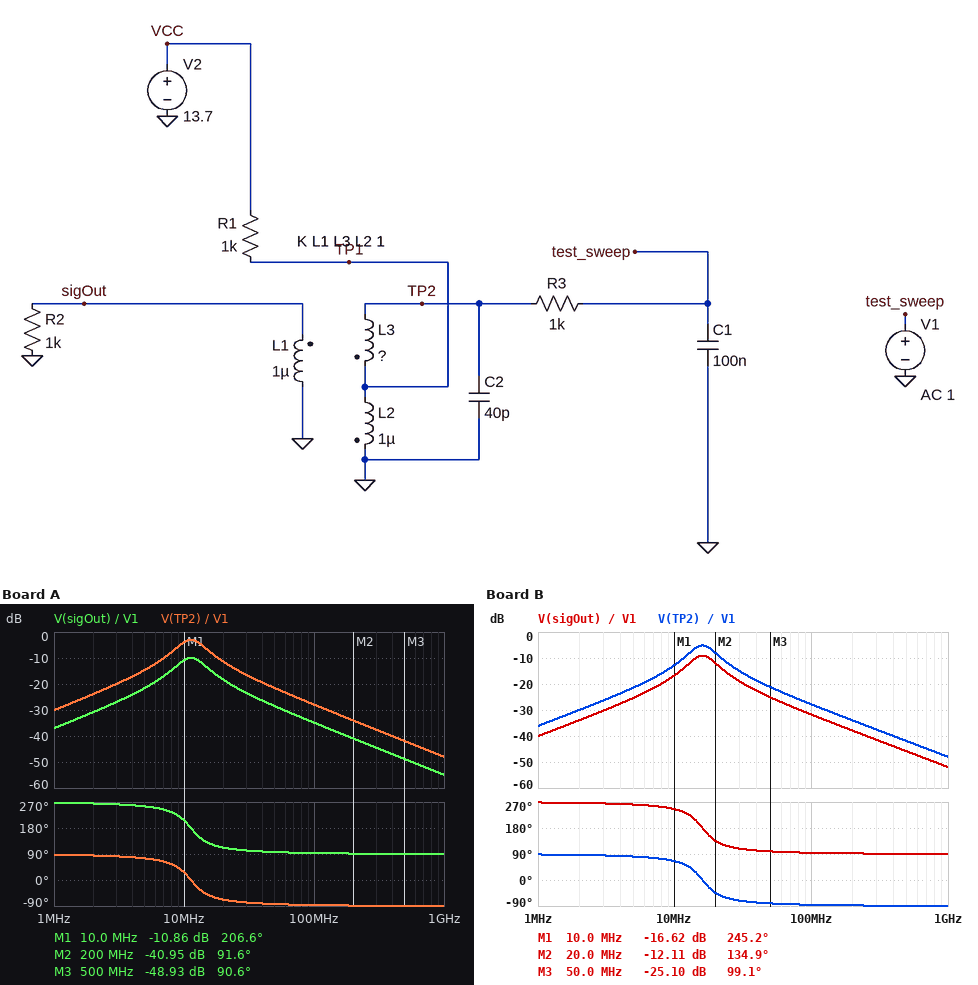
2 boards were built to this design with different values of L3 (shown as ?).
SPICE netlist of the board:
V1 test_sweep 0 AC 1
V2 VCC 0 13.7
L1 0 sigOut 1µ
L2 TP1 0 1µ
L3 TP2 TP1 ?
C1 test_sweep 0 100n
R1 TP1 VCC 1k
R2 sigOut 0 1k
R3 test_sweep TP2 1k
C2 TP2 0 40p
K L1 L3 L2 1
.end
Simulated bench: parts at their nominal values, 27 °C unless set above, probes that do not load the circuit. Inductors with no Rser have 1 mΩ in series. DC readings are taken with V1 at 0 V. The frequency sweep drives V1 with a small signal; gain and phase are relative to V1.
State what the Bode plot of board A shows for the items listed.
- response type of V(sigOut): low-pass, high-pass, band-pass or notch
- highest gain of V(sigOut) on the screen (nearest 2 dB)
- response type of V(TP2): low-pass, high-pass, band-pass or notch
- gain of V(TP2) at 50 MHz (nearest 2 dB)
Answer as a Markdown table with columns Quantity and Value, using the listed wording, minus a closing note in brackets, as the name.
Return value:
| Quantity | Value |
|---|---|
| response type of V(sigOut): low-pass, high-pass, band-pass or notch | band-pass |
| highest gain of V(sigOut) on the screen | -10 dB |
| response type of V(TP2): low-pass, high-pass, band-pass or notch | band-pass |
| gain of V(TP2) at 50 MHz | -22 dB |
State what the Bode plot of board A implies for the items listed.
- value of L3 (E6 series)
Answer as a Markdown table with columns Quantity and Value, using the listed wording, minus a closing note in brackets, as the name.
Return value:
| Quantity | Value |
|---|---|
| value of L3 | 1.5 µH |
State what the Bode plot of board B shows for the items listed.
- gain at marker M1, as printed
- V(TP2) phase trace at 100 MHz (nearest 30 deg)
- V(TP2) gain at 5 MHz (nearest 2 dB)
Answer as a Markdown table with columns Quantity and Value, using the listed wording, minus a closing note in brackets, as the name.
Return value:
| Quantity | Value |
|---|---|
| gain at marker M1, as printed | -16.62 dB |
| V(TP2) phase trace at 100 MHz | -90 deg |
| V(TP2) gain at 5 MHz | -22 dB |
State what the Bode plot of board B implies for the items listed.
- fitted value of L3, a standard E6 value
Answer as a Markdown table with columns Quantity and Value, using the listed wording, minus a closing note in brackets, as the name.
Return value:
| Quantity | Value |
|---|---|
| fitted value of L3, a standard E6 value | 330 nH |
